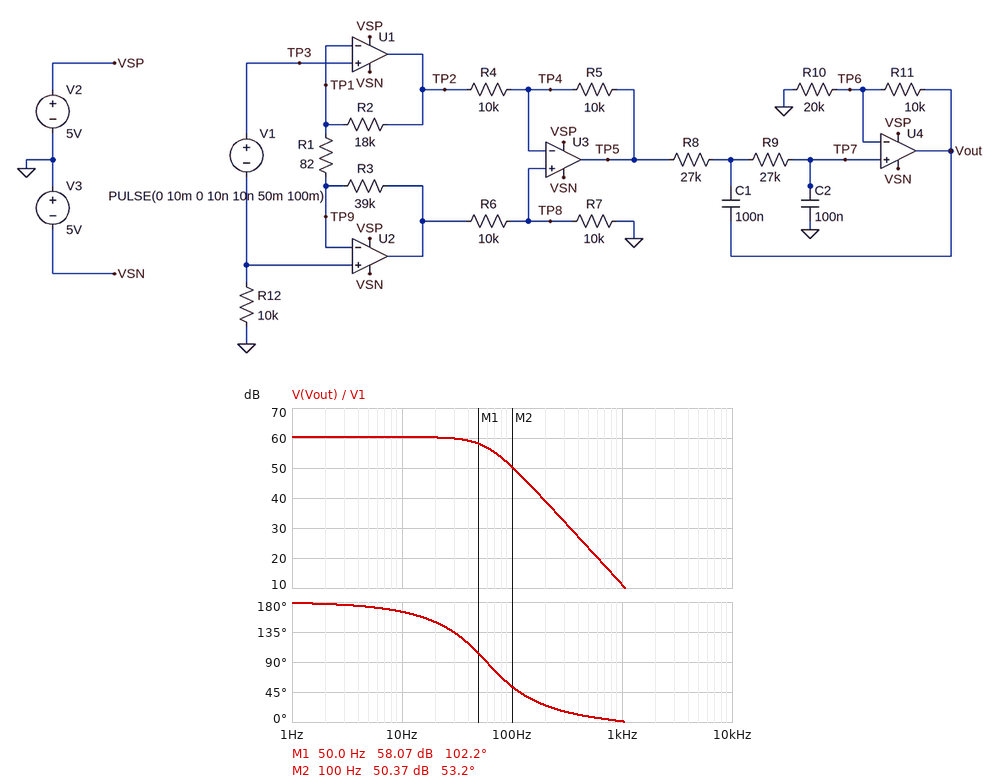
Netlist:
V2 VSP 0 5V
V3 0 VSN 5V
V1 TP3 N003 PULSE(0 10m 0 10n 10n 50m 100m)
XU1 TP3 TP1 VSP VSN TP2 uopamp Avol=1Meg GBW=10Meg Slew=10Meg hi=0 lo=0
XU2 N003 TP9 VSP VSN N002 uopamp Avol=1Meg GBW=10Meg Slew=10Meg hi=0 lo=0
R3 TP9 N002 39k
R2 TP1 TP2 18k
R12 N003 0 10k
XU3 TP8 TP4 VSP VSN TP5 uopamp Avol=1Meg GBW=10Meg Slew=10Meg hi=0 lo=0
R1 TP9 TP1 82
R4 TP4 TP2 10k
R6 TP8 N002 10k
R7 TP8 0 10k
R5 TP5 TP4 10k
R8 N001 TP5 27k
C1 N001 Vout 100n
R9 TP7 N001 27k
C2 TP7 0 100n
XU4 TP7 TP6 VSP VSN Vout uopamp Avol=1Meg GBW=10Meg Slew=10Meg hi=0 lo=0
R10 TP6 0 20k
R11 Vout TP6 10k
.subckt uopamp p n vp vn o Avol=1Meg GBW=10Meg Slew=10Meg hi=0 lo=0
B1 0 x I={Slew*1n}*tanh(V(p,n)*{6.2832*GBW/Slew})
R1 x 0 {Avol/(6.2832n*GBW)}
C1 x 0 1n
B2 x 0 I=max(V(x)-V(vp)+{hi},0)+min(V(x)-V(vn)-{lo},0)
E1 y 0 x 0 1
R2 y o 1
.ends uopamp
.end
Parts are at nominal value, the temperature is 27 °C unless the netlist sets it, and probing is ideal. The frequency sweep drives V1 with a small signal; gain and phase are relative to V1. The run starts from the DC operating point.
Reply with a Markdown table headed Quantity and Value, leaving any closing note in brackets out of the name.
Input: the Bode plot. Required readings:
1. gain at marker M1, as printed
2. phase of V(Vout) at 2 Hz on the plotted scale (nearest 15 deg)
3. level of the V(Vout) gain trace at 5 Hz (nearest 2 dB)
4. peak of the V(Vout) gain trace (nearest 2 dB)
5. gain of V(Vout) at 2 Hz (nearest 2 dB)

| Quantity | Value |
|---|---|
| gain at marker M1, as printed | 58.07 dB |
| phase of V(Vout) at 2 Hz on the plotted scale | 180 deg |
| level of the V(Vout) gain trace at 5 Hz | 60 dB |
| peak of the V(Vout) gain trace | 60 dB |
| gain of V(Vout) at 2 Hz | 60 dB |
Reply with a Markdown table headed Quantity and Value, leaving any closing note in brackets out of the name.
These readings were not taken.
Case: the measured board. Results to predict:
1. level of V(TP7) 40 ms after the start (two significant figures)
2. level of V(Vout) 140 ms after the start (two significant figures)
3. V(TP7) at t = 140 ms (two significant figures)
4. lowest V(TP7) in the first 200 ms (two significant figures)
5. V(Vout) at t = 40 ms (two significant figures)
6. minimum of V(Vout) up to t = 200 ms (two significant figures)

| Quantity | Value |
|---|---|
| level of V(TP7) 40 ms after the start | -5.0 V |
| level of V(Vout) 140 ms after the start | -5.0 V |
| V(TP7) at t = 140 ms | -5.0 V |
| lowest V(TP7) in the first 200 ms | -5.0 V |
| V(Vout) at t = 40 ms | -5.0 V |
| minimum of V(Vout) up to t = 200 ms | -5.0 V |
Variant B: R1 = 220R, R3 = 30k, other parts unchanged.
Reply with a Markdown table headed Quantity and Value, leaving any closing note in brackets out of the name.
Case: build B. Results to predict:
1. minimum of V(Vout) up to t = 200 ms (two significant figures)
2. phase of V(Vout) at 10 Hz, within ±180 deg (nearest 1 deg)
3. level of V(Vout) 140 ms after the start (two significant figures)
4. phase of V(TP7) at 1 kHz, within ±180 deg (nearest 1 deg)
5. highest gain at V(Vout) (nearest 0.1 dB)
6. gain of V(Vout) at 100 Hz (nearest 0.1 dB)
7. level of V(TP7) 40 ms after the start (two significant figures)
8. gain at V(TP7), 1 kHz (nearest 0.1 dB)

| Quantity | Value |
|---|---|
| minimum of V(Vout) up to t = 200 ms | -3.4 V |
| phase of V(Vout) at 10 Hz, within ±180 deg | 165 deg |
| level of V(Vout) 140 ms after the start | -3.3 V |
| phase of V(TP7) at 1 kHz, within ±180 deg | 4 deg |
| highest gain at V(Vout) | 50.3 dB |
| gain of V(Vout) at 100 Hz | 40.3 dB |
| level of V(TP7) 40 ms after the start | -2.2 V |
| gain at V(TP7), 1 kHz | -2.4 dB |
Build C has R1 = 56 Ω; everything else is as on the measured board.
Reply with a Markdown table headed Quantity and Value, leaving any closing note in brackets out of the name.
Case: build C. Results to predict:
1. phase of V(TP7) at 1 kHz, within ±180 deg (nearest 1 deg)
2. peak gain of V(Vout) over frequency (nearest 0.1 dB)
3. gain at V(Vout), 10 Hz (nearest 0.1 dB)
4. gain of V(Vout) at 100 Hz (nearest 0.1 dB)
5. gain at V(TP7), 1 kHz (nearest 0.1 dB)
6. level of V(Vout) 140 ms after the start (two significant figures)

| Quantity | Value |
|---|---|
| phase of V(TP7) at 1 kHz, within ±180 deg | -1 deg |
| peak gain of V(Vout) over frequency | 63.7 dB |
| gain at V(Vout), 10 Hz | 63.6 dB |
| gain of V(Vout) at 100 Hz | 53.7 dB |
| gain at V(TP7), 1 kHz | 10.9 dB |
| level of V(Vout) 140 ms after the start | -5.0 V |
